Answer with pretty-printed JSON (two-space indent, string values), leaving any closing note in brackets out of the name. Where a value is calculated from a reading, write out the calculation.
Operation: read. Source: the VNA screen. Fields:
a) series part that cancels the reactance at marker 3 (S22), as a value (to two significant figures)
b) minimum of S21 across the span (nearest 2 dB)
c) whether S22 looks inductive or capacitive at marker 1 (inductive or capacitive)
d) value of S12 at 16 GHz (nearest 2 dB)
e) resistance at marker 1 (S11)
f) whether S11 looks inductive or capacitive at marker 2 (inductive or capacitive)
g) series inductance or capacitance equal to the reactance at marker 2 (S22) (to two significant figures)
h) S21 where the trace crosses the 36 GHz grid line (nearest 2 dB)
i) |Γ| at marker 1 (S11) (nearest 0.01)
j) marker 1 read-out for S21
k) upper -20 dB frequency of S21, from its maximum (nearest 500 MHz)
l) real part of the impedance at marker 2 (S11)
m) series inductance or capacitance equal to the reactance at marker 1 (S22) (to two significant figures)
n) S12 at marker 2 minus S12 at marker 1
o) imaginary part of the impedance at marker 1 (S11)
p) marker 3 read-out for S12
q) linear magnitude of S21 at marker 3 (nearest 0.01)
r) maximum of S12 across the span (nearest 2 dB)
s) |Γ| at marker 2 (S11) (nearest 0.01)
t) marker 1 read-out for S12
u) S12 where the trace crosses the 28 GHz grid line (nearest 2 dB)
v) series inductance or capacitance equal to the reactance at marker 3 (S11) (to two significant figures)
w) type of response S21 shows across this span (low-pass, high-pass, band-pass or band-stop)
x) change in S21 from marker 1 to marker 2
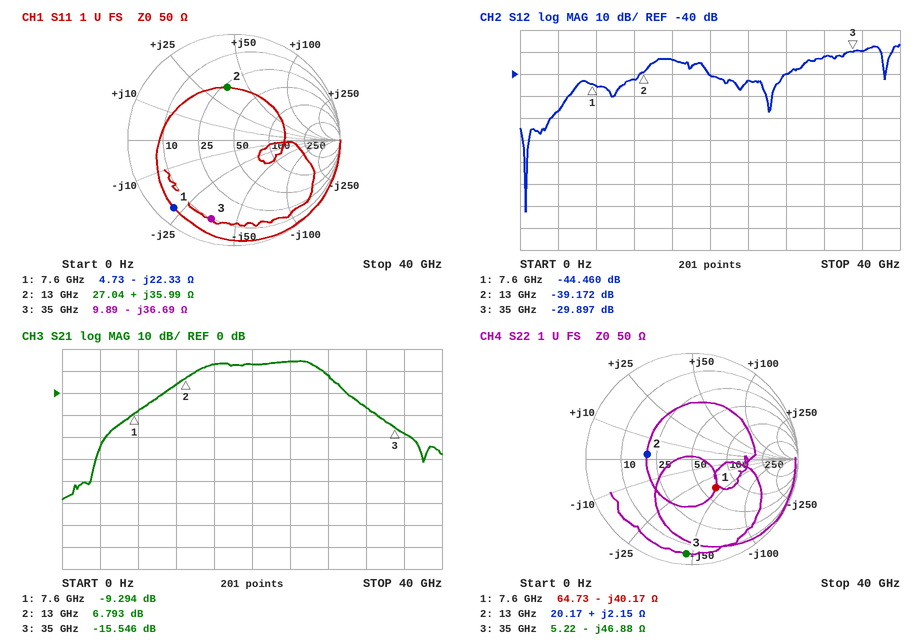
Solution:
{
  "series part that cancels the reactance at marker 3 (S22), as a value": "L = 46.88 Ω/(2π × 35 GHz) ≈ 213 pH, so 210 pH to two significant figures",
  "minimum of S21 across the span": "-48 dB",
  "whether S22 looks inductive or capacitive at marker 1": "capacitive",
  "value of S12 at 16 GHz": "-34 dB",
  "resistance at marker 1": "4.73 Ω",
  "whether S11 looks inductive or capacitive at marker 2": "inductive",
  "series inductance or capacitance equal to the reactance at marker 2 (S22)": "L = 2.15 Ω/(2π × 13 GHz) ≈ 26 pH",
  "S21 where the trace crosses the 36 GHz grid line": "-18 dB",
  "|Γ| at marker 1 (S11)": "0.85",
  "marker 1 read-out for S21": "-9.294 dB",
  "upper -20 dB frequency of S21, from its maximum": "31.5 GHz",
  "real part of the impedance at marker 2": "27.04 Ω",
  "series inductance or capacitance equal to the reactance at marker 1 (S22)": "C = 1/(2π × 7.6 GHz × 40.17 Ω) ≈ 521 fF, so 520 fF to two significant figures",
  "S12 at marker 2 minus S12 at marker 1": "-39.172 − (-44.46) = 5.288 dB",
  "imaginary part of the impedance at marker 1": "-22.33 Ω",
  "marker 3 read-out for S12": "-29.897 dB",
  "linear magnitude of S21 at marker 3": "10^(-15.546/20) ≈ 0.17",
  "maximum of S12 across the span": "-26 dB",
  "|Γ| at marker 2 (S11)": "0.50",
  "marker 1 read-out for S12": "-44.460 dB",
  "S12 where the trace crosses the 28 GHz grid line": "-40 dB",
  "series inductance or capacitance equal to the reactance at marker 3 (S11)": "C = 1/(2π × 35 GHz × 36.69 Ω) ≈ 124 fF, so 120 fF to two significant figures",
  "type of response S21 shows across this span": "band-pass",
  "change in S21 from marker 1 to marker 2": "6.793 − (-9.294) = 16.087 dB"
}
